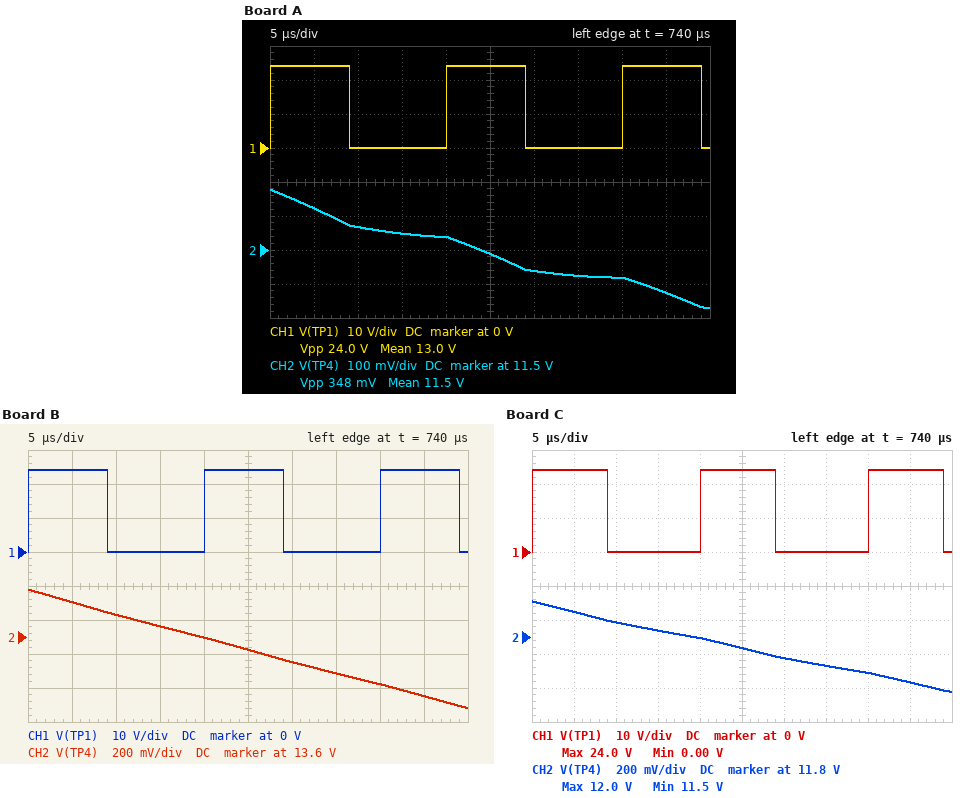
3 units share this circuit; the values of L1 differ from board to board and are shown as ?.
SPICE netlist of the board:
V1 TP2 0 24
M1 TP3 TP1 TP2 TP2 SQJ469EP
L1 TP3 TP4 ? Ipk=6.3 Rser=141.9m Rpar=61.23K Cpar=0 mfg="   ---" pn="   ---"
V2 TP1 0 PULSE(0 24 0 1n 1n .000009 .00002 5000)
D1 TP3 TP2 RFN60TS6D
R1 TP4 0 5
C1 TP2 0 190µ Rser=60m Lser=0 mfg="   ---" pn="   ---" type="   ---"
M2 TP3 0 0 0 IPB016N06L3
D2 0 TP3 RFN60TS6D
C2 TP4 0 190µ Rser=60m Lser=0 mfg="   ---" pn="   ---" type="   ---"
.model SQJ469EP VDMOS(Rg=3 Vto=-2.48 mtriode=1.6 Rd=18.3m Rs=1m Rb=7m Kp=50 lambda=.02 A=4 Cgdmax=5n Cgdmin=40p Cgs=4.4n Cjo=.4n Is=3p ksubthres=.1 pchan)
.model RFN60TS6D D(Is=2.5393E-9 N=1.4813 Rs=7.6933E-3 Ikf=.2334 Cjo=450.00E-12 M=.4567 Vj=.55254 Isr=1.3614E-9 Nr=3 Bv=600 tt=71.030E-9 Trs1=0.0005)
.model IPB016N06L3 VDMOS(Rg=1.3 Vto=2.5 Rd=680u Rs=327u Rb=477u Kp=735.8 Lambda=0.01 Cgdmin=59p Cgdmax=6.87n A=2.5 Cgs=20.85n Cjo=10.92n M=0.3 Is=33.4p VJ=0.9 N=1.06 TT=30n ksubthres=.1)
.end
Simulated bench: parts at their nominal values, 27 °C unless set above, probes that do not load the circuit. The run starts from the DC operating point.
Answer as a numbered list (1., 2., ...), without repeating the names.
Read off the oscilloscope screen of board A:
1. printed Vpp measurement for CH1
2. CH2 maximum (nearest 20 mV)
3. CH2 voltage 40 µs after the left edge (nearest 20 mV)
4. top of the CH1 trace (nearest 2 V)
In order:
1. 24.0 V
2. 11.68 V
3. 11.42 V
4. 24 V
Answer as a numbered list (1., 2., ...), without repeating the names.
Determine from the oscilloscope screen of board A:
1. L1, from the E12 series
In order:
1. 180 µH
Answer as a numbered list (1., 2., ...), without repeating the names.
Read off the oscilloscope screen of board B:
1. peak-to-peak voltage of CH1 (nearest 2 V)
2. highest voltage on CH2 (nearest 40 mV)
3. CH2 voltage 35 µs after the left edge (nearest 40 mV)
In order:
1. 24 V
2. 13.88 V
3. 13.40 V
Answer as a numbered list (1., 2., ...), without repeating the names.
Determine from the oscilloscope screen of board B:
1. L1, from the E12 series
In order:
1. 1 mH
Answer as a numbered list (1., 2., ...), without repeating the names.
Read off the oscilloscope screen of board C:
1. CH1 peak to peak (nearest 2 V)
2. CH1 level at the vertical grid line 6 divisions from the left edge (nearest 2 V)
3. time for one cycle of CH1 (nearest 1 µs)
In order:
1. 24 V
2. 0 V
3. 20 µs
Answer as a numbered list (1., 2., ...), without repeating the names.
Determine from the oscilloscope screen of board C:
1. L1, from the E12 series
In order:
1. 470 µH
